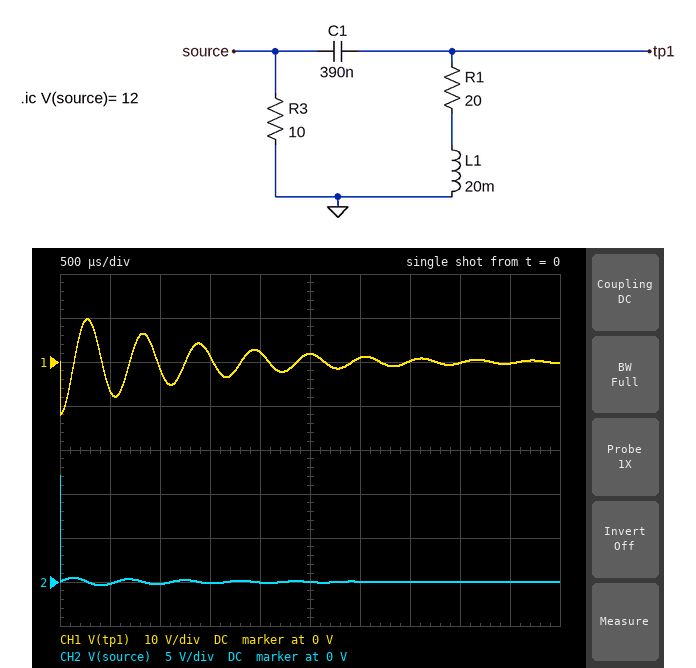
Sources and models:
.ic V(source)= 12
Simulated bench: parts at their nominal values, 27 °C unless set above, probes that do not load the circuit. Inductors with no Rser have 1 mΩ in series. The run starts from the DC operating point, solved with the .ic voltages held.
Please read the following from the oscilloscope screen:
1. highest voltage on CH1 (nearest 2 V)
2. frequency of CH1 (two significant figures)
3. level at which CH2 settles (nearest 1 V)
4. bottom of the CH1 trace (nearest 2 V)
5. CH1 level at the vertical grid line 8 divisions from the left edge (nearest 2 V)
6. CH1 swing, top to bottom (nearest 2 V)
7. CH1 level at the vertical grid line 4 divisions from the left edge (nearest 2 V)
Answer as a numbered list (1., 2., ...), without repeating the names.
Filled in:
1. 10 V
2. 1.8 kHz
3. 0 V
4. -12 V
5. 0 V
6. 22 V
7. 2 V
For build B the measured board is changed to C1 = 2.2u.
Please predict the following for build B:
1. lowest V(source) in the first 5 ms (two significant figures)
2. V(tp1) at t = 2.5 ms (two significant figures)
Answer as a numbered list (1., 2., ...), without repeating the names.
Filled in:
1. -610 mV
2. -1.2 V
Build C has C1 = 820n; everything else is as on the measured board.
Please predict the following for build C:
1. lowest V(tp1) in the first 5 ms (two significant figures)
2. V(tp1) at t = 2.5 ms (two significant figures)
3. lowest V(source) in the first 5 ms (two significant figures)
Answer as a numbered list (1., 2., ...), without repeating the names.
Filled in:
1. -12 V
2. -1.6 V
3. -490 mV
